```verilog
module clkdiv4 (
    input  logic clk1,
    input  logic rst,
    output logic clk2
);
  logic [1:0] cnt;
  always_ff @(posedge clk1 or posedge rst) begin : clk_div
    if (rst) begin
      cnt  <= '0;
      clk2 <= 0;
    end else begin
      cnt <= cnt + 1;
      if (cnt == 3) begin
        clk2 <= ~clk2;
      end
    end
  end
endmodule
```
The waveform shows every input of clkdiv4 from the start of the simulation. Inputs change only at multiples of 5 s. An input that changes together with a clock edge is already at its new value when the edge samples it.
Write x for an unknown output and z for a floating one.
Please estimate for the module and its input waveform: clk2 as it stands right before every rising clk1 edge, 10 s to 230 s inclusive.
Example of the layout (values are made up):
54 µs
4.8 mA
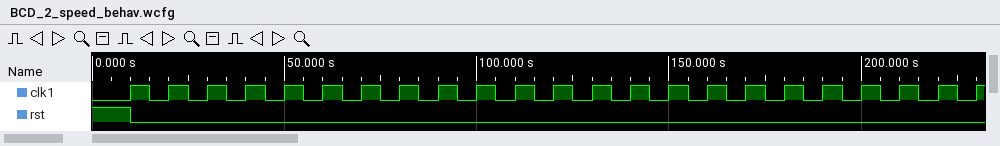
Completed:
0 0 0 0 1 1 1 1 0 0 0 0 1 1 1 1 0 0 0 0 1 1 1
